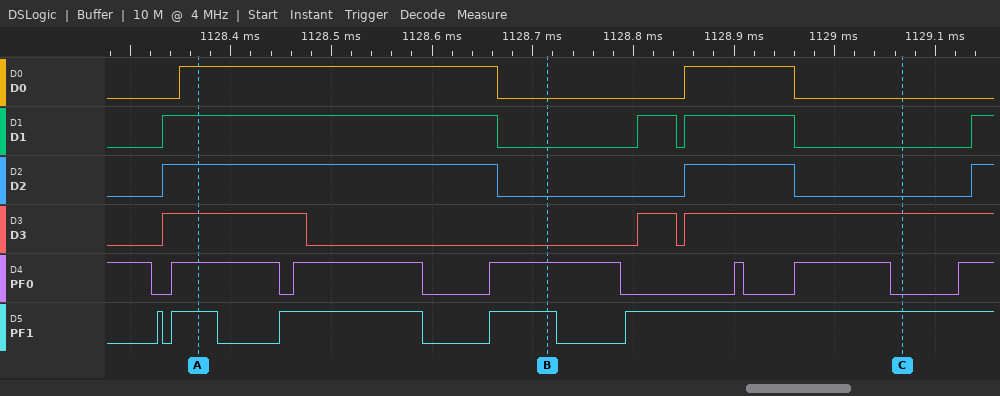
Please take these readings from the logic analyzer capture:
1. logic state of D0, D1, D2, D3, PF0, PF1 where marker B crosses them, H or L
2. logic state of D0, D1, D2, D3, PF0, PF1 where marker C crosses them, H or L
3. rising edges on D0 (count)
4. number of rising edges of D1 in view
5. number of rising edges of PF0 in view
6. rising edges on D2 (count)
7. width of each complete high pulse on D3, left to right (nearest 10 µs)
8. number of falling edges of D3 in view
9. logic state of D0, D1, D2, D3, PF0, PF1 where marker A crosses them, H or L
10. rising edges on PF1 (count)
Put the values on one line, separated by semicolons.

D0=L, D1=L, D2=L, D3=L, PF0=H, PF1=H; D0=L, D1=L, D2=L, D3=H, PF0=L, PF1=H; 2; 4; 6; 3; 140 µs, 40 µs; 2; D0=H, D1=H, D2=H, D3=H, PF0=H, PF1=H; 5
